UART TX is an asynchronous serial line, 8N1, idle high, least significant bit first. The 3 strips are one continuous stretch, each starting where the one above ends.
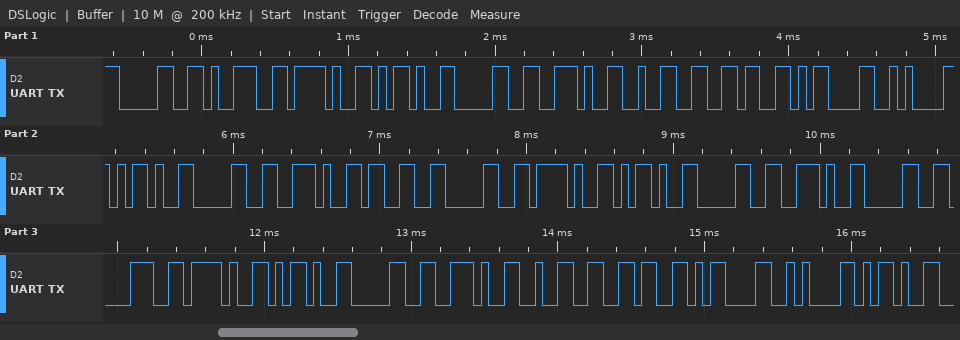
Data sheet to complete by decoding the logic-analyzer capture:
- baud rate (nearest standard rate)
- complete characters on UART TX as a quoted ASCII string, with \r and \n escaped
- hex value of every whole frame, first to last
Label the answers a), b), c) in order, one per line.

a) 19200 baud
b) "09/-0.26\r\n-0.30/-0.08/-0.26\r\n-"
c) 0x30 0x39 0x2F 0x2D 0x30 0x2E 0x32 0x36 0x0D 0x0A 0x2D 0x30 0x2E 0x33 0x30 0x2F 0x2D 0x30 0x2E 0x30 0x38 0x2F 0x2D 0x30 0x2E 0x32 0x36 0x0D 0x0A 0x2D
